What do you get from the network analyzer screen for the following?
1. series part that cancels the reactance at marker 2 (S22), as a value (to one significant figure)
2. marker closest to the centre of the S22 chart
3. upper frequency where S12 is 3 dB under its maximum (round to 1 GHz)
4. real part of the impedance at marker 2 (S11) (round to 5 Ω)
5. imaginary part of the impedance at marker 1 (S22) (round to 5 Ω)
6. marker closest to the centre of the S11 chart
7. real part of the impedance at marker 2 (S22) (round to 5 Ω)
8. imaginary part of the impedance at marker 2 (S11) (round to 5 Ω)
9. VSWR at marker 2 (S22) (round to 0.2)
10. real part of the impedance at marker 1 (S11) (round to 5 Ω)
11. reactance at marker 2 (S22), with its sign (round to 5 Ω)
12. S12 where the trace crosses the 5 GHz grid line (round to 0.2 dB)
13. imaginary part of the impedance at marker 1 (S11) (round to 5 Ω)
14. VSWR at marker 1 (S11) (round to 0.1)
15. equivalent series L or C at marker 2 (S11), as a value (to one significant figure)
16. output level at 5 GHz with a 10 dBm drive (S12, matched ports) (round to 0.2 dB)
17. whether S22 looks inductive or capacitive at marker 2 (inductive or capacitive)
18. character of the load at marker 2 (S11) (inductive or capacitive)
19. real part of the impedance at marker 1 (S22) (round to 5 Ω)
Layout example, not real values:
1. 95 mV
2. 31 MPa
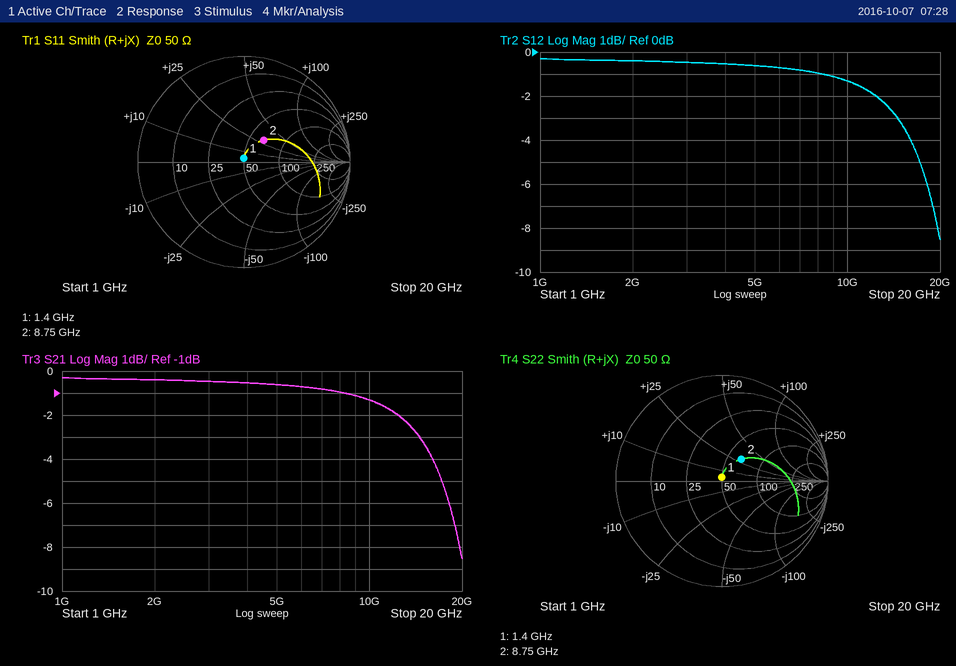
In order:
1. 600 fF
2. marker 1
3. 15 GHz
4. 65 Ω
5. +5 Ω
6. marker 1
7. 65 Ω
8. +30 Ω
9. 1.8
10. 50 Ω
11. +30 Ω
12. -0.6 dB
13. +5 Ω
14. 1.1
15. 500 pH
16. 9.4 dBm
17. inductive
18. inductive
19. 50 Ω
